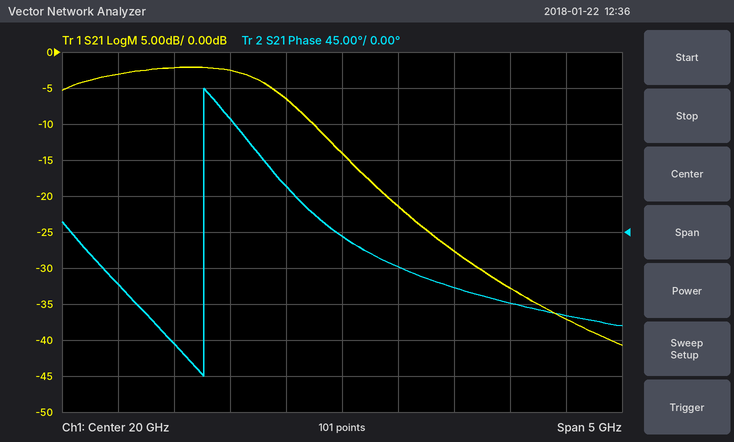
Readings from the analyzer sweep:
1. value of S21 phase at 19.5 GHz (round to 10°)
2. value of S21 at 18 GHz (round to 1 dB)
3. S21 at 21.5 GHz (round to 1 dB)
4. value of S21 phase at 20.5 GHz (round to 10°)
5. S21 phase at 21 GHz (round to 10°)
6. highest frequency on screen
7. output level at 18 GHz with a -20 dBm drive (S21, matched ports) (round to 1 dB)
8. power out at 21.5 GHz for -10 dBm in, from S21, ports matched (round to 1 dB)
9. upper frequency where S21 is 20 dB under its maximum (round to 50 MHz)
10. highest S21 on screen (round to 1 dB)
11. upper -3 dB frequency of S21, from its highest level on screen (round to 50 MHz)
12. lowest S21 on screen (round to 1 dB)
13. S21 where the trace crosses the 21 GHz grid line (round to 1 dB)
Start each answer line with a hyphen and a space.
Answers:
- 60°
- -3 dB
- -33 dB
- -40°
- -70°
- 22.5 GHz
- -23 dBm
- -43 dBm
- 20.55 GHz
- -2 dB
- 19.40 GHz
- -41 dB
- -28 dB
